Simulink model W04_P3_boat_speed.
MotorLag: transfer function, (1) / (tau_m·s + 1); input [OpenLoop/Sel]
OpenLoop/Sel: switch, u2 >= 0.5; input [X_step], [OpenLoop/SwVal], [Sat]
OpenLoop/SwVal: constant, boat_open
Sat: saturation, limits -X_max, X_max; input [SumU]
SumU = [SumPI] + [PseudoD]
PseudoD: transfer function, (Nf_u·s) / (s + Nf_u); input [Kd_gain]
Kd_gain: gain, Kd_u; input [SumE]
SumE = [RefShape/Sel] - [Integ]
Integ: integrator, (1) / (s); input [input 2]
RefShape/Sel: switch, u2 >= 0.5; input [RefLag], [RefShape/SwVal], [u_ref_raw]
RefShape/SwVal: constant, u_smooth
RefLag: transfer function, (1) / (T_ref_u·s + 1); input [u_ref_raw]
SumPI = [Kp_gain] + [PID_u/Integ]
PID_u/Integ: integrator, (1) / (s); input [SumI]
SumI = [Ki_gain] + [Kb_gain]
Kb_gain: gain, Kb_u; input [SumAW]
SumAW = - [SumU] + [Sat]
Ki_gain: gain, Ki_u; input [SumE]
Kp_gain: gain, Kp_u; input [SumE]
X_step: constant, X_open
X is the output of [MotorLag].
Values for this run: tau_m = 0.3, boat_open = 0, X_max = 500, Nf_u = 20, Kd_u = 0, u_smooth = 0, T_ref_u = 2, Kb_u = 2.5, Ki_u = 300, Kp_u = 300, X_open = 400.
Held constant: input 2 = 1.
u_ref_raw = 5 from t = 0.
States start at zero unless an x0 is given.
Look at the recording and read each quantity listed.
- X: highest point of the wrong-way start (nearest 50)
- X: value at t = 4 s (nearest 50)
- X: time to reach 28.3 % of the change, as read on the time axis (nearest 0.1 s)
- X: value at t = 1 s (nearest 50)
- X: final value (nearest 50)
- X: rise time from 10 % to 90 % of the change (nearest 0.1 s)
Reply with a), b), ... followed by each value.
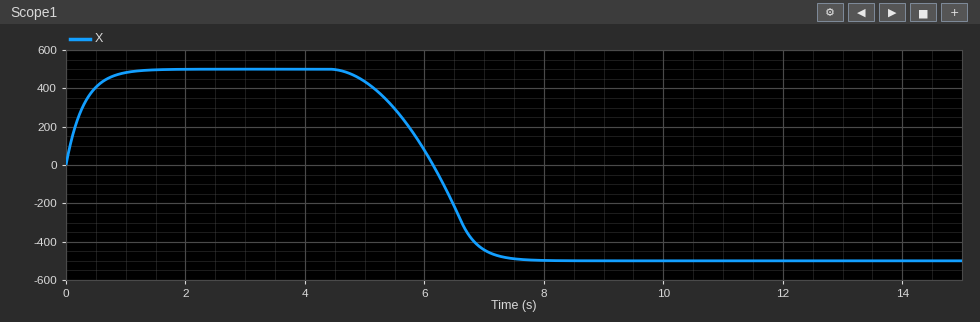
a) 500
b) 500
c) 6.4 s
d) 500
e) -500
f) 0.8 s
